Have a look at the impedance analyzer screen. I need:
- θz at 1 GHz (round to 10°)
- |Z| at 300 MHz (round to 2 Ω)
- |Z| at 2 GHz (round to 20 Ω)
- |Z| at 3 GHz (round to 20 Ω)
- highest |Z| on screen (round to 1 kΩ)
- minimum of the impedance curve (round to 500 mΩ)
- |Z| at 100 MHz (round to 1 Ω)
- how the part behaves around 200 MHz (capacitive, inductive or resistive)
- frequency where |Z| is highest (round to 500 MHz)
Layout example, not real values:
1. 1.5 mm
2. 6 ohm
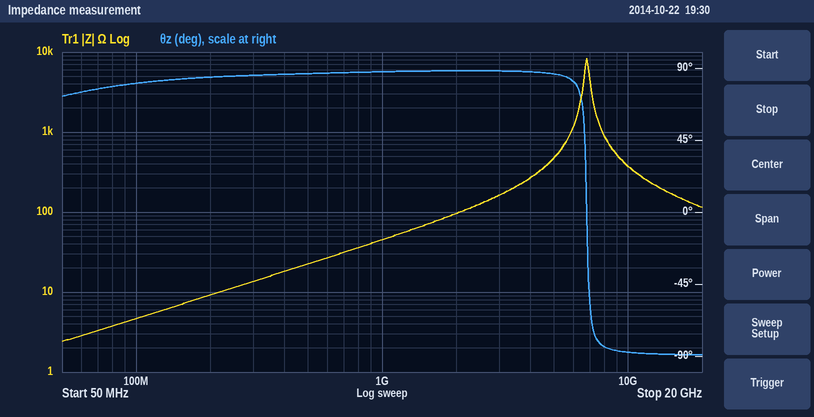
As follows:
1. 90°
2. 14 Ω
3. 100 Ω
4. 160 Ω
5. 8 kΩ
6. 2.5 Ω
7. 5 Ω
8. inductive
9. 7.0 GHz
